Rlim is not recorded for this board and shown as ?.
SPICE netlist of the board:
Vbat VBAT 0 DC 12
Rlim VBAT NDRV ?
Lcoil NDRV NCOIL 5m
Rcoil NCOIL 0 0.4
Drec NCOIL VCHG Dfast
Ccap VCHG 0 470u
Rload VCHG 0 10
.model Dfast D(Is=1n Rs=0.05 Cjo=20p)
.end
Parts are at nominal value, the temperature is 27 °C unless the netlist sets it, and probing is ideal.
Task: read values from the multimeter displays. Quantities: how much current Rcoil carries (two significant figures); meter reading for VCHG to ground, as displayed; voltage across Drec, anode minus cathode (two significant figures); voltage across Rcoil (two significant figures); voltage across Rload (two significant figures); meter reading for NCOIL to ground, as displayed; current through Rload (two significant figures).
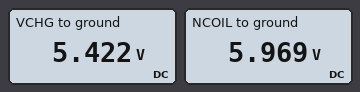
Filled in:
15 A
5.422 V
550 mV
6.0 V
5.4 V
5.969 V
540 mA
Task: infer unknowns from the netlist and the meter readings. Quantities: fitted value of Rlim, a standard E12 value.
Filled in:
0.39 Ω
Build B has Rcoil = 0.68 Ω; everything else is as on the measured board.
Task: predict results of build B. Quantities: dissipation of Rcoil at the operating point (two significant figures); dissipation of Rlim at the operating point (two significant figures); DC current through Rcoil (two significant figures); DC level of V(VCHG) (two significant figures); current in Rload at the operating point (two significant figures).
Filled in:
82 W
53 W
11 A
6.9 V
690 mA
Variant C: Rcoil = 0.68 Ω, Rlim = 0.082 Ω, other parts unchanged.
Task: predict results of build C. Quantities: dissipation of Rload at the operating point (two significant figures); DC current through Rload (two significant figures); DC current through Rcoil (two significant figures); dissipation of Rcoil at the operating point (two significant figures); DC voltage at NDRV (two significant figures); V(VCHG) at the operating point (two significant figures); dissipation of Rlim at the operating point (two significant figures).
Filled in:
10 W
1.0 A
16 A
170 W
11 V
10 V
23 W
